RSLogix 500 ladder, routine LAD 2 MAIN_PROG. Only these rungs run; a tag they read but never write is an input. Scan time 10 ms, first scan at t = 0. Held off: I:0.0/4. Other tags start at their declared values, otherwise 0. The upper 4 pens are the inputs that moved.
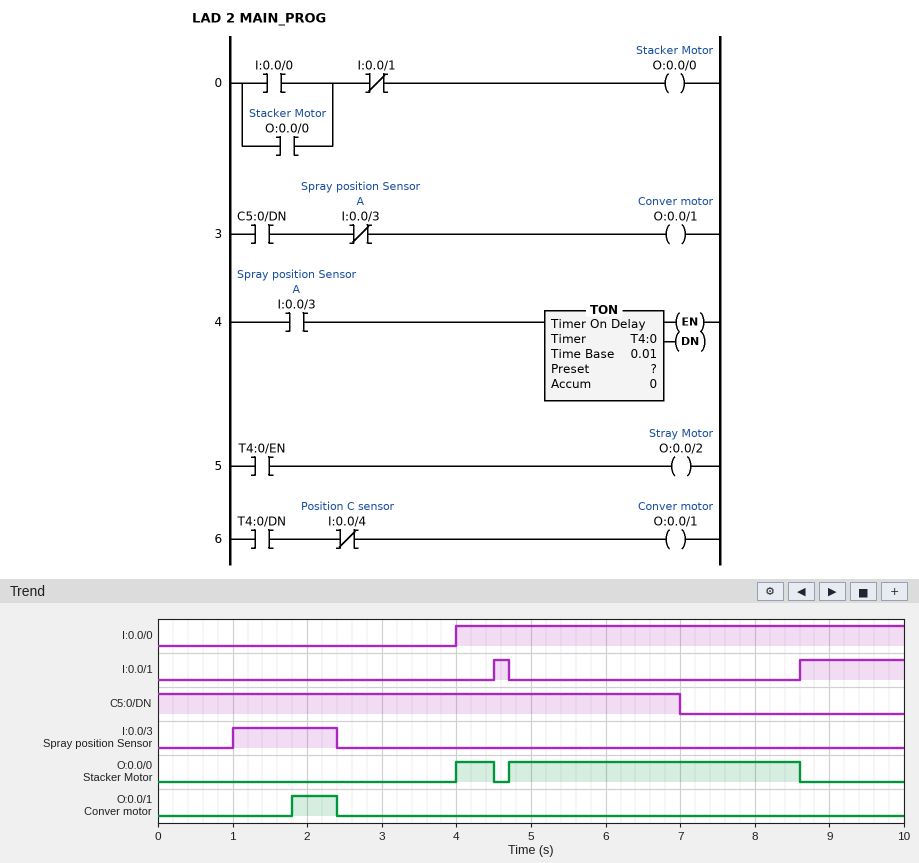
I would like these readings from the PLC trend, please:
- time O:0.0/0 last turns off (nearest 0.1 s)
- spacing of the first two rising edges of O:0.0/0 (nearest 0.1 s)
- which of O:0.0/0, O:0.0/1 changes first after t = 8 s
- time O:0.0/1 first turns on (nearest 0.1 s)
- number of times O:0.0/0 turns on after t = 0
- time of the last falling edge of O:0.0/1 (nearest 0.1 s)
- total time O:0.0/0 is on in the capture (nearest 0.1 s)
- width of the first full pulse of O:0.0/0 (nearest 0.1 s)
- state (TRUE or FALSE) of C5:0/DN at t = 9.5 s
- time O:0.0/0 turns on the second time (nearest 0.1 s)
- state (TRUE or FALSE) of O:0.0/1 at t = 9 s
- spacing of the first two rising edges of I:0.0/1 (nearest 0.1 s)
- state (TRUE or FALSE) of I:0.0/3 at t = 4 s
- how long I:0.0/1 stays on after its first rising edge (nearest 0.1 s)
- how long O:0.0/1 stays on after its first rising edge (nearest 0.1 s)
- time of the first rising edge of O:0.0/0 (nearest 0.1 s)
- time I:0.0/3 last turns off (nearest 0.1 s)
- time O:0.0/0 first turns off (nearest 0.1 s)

8.6 s
0.7 s
O:0.0/0
1.8 s
2
2.4 s
4.4 s
0.5 s
FALSE
4.7 s
FALSE
4.1 s
FALSE
0.2 s
0.6 s
4.0 s
2.4 s
4.5 s
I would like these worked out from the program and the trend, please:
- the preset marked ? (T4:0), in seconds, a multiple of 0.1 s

0.8 s
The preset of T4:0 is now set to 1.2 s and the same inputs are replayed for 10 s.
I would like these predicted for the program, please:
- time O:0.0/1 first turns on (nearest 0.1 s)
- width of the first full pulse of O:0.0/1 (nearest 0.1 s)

2.2 s
0.2 s
